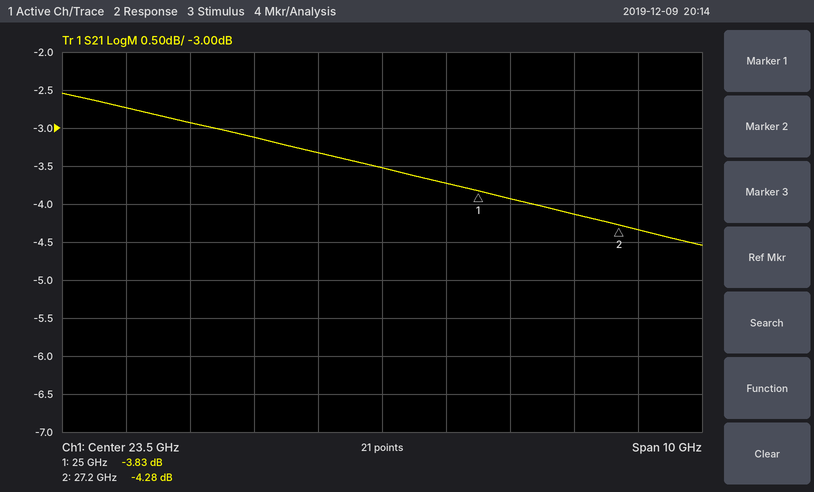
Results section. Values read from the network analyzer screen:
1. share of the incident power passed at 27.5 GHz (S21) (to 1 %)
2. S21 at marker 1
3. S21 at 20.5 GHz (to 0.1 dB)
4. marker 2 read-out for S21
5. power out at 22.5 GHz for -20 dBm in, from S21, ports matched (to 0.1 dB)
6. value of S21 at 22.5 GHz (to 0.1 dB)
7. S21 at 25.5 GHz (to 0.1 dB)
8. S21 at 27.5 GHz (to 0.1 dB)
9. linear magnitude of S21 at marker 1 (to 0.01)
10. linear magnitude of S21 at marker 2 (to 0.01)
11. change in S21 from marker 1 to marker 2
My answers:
37 %
-3.83 dB
-2.9 dB
-4.28 dB
-23.3 dBm
-3.3 dB
-3.9 dB
-4.3 dB
0.64
0.61
-0.45 dB
